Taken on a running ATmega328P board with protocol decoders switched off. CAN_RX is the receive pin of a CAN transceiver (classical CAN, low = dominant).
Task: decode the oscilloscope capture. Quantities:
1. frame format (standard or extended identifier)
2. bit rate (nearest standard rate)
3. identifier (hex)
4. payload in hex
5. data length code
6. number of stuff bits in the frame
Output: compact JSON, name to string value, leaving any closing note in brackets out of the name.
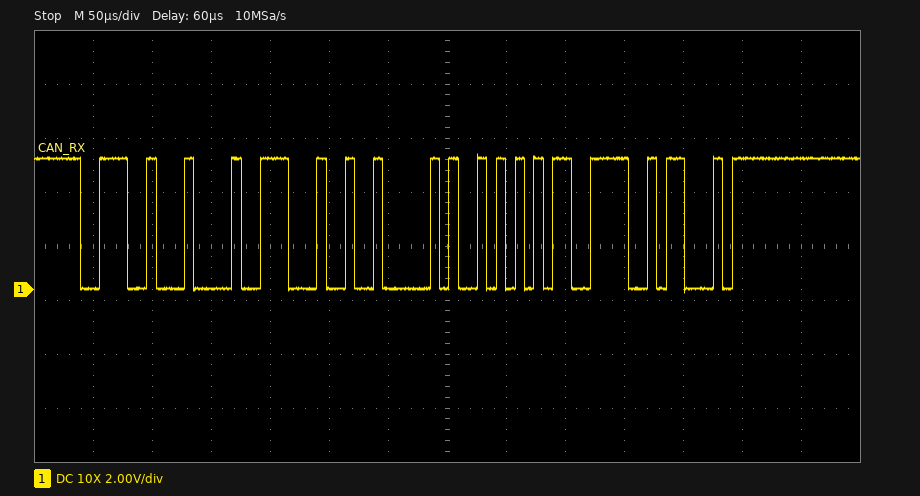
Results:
{"frame format": "standard", "bit rate": "125 kbit/s", "identifier": "0x391", "payload in hex": "E2 48 12 AB", "data length code": "4", "number of stuff bits in the frame": "1"}
